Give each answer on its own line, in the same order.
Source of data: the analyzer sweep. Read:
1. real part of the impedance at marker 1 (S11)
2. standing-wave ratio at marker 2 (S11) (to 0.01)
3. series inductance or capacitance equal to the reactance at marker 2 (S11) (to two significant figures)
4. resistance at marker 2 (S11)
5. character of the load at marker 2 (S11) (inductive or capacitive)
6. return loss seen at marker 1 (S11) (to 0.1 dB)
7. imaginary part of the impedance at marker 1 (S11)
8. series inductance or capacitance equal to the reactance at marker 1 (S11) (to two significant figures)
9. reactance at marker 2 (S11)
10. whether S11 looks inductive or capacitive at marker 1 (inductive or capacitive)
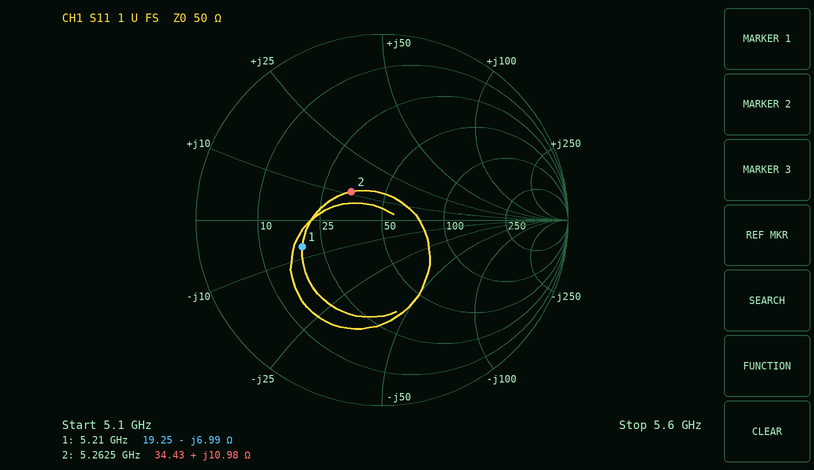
19.25 Ω
1.58
330 pH
34.43 Ω
inductive
6.9 dB
-6.99 Ω
4.4 pF
+10.98 Ω
capacitive
